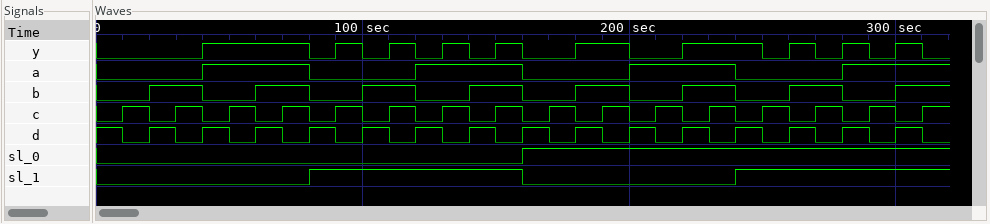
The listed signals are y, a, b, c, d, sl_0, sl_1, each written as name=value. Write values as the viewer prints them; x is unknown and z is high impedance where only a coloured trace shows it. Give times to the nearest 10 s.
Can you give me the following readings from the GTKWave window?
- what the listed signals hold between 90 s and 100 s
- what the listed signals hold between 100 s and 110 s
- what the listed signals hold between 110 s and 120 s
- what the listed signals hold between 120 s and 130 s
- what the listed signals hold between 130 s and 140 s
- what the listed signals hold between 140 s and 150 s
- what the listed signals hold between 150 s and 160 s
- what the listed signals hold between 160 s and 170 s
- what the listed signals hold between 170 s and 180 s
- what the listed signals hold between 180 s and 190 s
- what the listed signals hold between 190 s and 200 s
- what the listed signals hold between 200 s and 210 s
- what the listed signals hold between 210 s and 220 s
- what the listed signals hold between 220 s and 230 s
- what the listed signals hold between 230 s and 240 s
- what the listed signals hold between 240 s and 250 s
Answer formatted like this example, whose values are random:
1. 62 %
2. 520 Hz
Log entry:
1. y=1, a=0, b=0, c=1, d=0, sl_0=0, sl_1=1
2. y=0, a=0, b=1, c=0, d=1, sl_0=0, sl_1=1
3. y=1, a=0, b=1, c=1, d=0, sl_0=0, sl_1=1
4. y=0, a=1, b=0, c=0, d=1, sl_0=0, sl_1=1
5. y=1, a=1, b=0, c=1, d=0, sl_0=0, sl_1=1
6. y=0, a=1, b=1, c=0, d=1, sl_0=0, sl_1=1
7. y=1, a=1, b=1, c=1, d=0, sl_0=0, sl_1=1
8. y=0, a=0, b=0, c=0, d=1, sl_0=1, sl_1=0
9. y=0, a=0, b=0, c=1, d=0, sl_0=1, sl_1=0
10. y=1, a=0, b=1, c=0, d=1, sl_0=1, sl_1=0
11. y=1, a=0, b=1, c=1, d=0, sl_0=1, sl_1=0
12. y=0, a=1, b=0, c=0, d=1, sl_0=1, sl_1=0
13. y=0, a=1, b=0, c=1, d=0, sl_0=1, sl_1=0
14. y=1, a=1, b=1, c=0, d=1, sl_0=1, sl_1=0
15. y=1, a=1, b=1, c=1, d=0, sl_0=1, sl_1=0
16. y=1, a=0, b=0, c=0, d=1, sl_0=1, sl_1=1
